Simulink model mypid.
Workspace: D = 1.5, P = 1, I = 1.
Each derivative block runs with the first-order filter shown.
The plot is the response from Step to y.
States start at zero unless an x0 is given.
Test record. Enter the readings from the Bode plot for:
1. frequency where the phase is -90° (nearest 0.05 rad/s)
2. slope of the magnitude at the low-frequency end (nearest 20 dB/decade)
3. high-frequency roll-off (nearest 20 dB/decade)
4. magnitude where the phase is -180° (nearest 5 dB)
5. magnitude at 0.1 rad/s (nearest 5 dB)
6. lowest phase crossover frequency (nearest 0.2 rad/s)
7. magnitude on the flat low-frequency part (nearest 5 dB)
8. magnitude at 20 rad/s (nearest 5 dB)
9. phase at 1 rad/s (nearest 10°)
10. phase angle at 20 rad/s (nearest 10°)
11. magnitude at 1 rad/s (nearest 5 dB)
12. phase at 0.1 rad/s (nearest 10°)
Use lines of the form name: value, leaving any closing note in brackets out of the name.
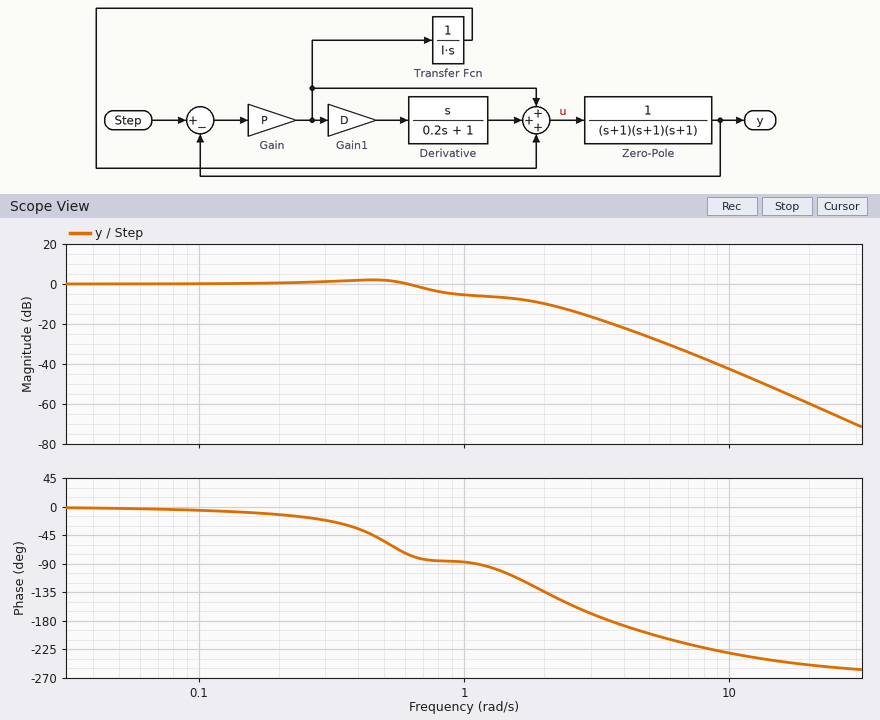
frequency where the phase is -90°: 1.10 rad/s
slope of the magnitude at the low-frequency end: 0 dB/decade
high-frequency roll-off: -60 dB/decade
magnitude where the phase is -180°: -20 dB
magnitude at 0.1 rad/s: 0 dB
lowest phase crossover frequency: 3.6 rad/s
magnitude on the flat low-frequency part: 0 dB
magnitude at 20 rad/s: -60 dB
phase at 1 rad/s: -90°
phase angle at 20 rad/s: -250°
magnitude at 1 rad/s: -5 dB
phase at 0.1 rad/s: -10°
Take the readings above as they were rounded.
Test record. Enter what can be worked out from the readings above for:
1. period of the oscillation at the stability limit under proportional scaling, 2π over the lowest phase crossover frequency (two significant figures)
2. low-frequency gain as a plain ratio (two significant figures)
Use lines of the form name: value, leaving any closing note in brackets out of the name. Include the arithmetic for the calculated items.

period of the oscillation at the stability limit under proportional scaling, 2π over the lowest phase crossover frequency: 2π / 3.6 = 1.7 s
low-frequency gain as a plain ratio: 10^(0 / 20) = 1.0
